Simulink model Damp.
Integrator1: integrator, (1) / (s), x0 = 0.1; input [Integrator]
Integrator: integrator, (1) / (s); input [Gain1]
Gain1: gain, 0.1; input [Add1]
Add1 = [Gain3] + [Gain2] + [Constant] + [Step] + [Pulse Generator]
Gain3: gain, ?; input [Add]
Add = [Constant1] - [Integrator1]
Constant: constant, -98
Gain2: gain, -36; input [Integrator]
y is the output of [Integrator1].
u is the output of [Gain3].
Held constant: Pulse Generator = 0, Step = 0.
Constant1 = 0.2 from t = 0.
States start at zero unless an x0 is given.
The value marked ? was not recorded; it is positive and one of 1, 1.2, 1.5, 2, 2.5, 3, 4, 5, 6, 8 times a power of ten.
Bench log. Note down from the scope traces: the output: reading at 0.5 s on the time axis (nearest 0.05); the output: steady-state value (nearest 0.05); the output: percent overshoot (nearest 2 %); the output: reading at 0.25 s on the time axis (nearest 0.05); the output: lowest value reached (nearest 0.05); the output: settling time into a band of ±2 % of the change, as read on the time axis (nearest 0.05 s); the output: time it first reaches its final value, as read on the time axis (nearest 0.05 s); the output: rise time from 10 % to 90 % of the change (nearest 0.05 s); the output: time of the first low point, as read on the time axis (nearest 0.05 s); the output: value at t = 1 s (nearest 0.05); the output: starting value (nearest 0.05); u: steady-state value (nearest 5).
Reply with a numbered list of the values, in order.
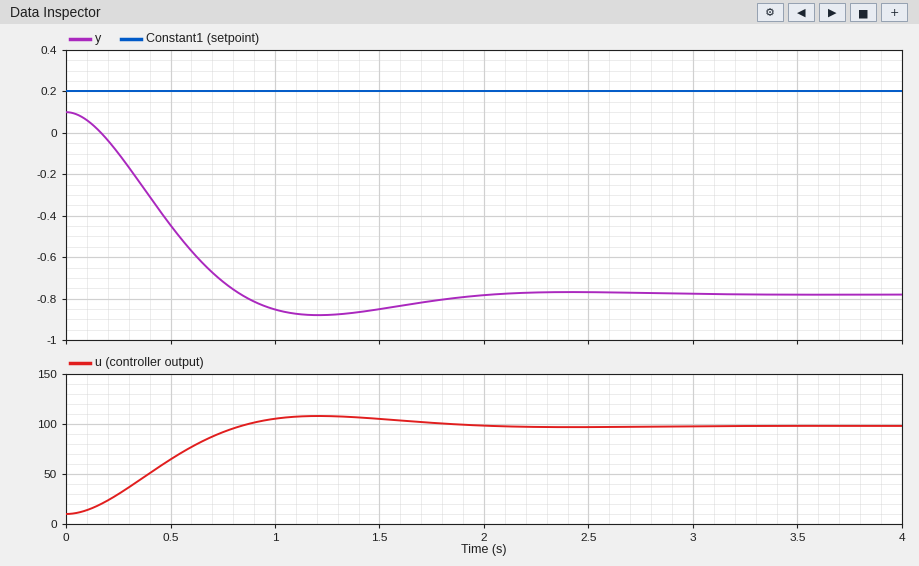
1. -0.45
2. -0.80
3. 12 %
4. -0.10
5. -0.90
6. 1.85 s
7. 0.85 s
8. 0.55 s
9. 1.20 s
10. -0.85
11. 0.10
12. 100
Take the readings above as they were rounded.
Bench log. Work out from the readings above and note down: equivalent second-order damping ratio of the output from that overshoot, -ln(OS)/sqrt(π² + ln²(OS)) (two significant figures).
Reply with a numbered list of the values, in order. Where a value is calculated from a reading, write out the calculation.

1. ln(0.12) = -2.120; 2.120 / sqrt(9.870 + 4.496) = 0.56
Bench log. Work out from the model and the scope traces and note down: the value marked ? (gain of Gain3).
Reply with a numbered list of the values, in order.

1. 100
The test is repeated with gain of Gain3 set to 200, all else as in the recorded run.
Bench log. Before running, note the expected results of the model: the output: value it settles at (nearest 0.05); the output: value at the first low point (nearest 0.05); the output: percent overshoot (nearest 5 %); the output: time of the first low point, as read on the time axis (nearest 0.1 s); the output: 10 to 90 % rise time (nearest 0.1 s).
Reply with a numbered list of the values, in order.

1. -0.30
2. -0.40
3. 25 %
4. 0.8 s
5. 0.3 s
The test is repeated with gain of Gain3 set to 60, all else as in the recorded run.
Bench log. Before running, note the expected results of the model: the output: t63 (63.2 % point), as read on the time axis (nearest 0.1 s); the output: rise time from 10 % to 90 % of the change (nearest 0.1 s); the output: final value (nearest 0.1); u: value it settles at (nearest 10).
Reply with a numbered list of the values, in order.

1. 0.7 s
2. 0.9 s
3. -1.4
4. 100
